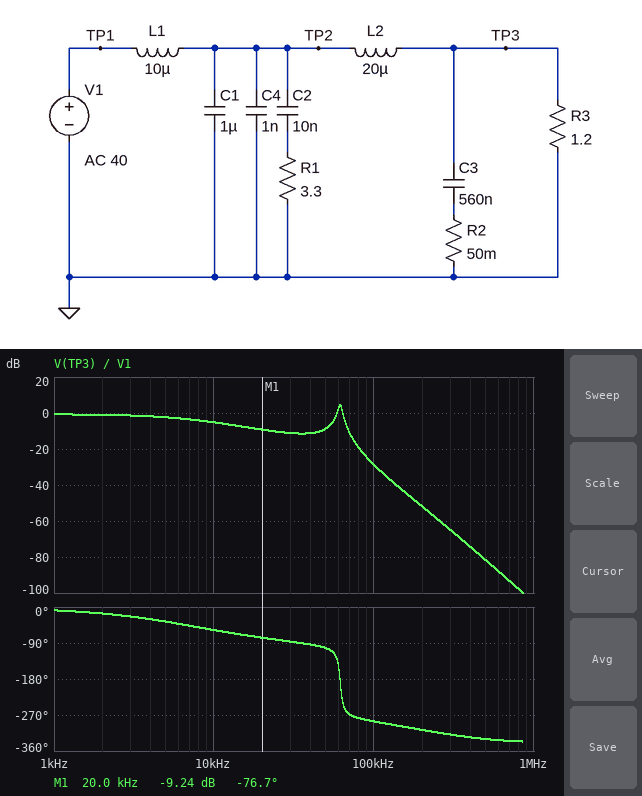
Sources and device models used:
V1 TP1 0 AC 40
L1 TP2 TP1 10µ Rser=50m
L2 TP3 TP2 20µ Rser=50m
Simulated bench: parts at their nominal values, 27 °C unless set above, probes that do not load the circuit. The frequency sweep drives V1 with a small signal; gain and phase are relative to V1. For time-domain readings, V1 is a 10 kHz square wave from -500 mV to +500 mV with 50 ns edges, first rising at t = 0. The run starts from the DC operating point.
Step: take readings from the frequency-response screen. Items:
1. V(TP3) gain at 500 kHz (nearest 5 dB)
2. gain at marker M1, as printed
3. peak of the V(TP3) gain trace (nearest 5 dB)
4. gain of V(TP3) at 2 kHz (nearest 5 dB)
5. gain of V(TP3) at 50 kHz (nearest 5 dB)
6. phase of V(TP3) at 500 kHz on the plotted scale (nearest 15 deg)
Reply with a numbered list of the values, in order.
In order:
1. -80 dB
2. -9.24 dB
3. 5 dB
4. 0 dB
5. -10 dB
6. -330 deg
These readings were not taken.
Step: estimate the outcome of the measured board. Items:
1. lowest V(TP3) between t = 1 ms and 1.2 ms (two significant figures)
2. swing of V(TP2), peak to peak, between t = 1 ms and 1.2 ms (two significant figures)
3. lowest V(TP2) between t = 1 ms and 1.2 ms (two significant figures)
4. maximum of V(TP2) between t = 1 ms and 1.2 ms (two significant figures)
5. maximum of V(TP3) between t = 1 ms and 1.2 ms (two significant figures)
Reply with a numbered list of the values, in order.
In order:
1. -390 mV
2. 1.4 V
3. -720 mV
4. 720 mV
5. 390 mV
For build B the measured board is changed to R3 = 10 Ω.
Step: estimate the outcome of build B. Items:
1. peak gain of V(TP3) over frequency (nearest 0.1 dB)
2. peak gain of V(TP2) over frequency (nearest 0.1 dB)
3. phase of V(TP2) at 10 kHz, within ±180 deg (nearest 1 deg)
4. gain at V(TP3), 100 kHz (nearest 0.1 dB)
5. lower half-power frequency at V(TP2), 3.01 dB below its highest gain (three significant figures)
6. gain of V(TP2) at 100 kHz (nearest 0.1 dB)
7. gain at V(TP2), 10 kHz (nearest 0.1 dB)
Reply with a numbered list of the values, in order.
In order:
1. 9.0 dB
2. 11.6 dB
3. -4 deg
4. -18.8 dB
5. 63.8 kHz
6. -7.5 dB
7. 0.4 dB
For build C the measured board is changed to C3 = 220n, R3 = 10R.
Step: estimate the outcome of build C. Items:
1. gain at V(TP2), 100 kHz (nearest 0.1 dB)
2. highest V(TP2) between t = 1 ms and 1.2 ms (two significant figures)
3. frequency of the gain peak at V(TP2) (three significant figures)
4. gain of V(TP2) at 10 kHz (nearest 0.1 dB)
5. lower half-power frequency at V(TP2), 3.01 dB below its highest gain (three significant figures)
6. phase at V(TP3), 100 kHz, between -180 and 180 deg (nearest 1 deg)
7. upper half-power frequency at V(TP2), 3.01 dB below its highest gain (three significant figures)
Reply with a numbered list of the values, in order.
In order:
1. -7.4 dB
2. 1.0 V
3. 48.2 kHz
4. 0.3 dB
5. 32.2 kHz
6. 68 deg
7. 64.0 kHz
